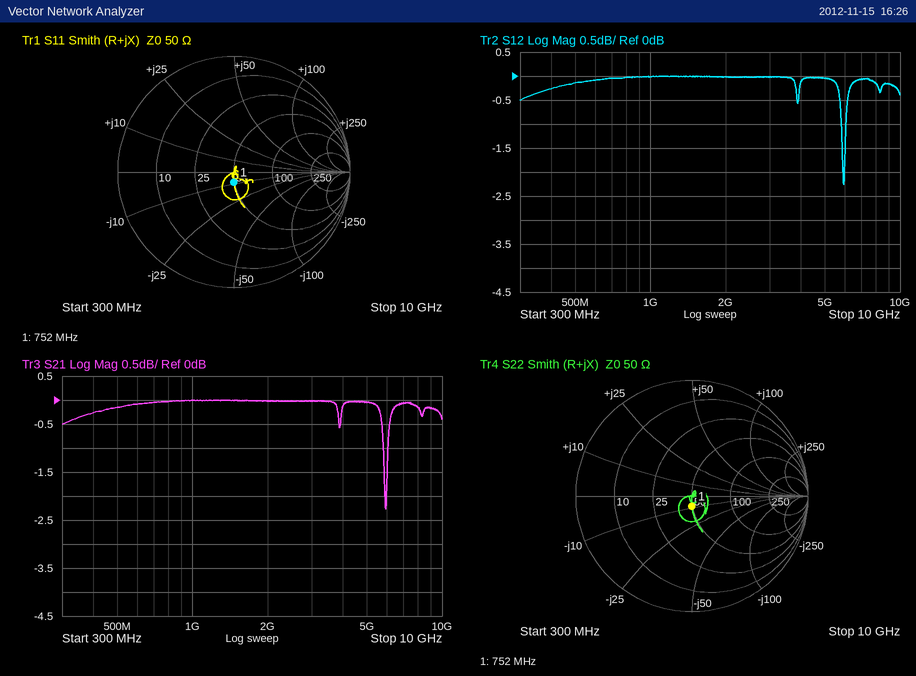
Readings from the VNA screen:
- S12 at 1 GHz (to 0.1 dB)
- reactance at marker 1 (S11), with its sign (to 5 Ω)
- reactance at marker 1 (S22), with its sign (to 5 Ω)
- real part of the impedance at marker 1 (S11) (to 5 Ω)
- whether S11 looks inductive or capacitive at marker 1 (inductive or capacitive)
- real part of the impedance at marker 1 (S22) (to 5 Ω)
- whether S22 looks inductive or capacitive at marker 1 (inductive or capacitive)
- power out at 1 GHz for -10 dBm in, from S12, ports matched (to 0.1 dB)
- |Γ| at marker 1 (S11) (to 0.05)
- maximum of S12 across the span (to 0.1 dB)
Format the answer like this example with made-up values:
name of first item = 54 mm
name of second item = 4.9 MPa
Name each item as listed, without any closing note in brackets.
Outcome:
S12 at 1 GHz = 0.0 dB
reactance at marker 1 (S11), with its sign = -10 Ω
reactance at marker 1 (S22), with its sign = -10 Ω
real part of the impedance at marker 1 (S11) = 50 Ω
whether S11 looks inductive or capacitive at marker 1 = capacitive
real part of the impedance at marker 1 (S22) = 50 Ω
whether S22 looks inductive or capacitive at marker 1 = capacitive
power out at 1 GHz for -10 dBm in, from S12, ports matched = -10.0 dBm
|Γ| at marker 1 (S11) = 0.10
maximum of S12 across the span = 0.0 dB
